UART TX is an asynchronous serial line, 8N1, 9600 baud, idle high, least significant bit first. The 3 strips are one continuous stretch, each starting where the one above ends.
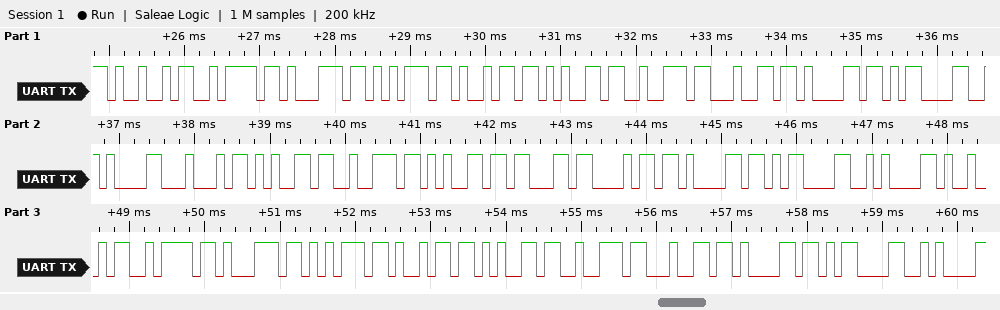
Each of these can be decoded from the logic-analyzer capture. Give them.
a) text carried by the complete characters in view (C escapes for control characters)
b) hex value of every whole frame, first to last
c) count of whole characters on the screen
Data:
"Izquierda\r\nDerecha\r\nIzquierda\r\n"
49 7A 71 75 69 65 72 64 61 0D 0A 44 65 72 65 63 68 61 0D 0A 49 7A 71 75 69 65 72 64 61 0D 0A
31
